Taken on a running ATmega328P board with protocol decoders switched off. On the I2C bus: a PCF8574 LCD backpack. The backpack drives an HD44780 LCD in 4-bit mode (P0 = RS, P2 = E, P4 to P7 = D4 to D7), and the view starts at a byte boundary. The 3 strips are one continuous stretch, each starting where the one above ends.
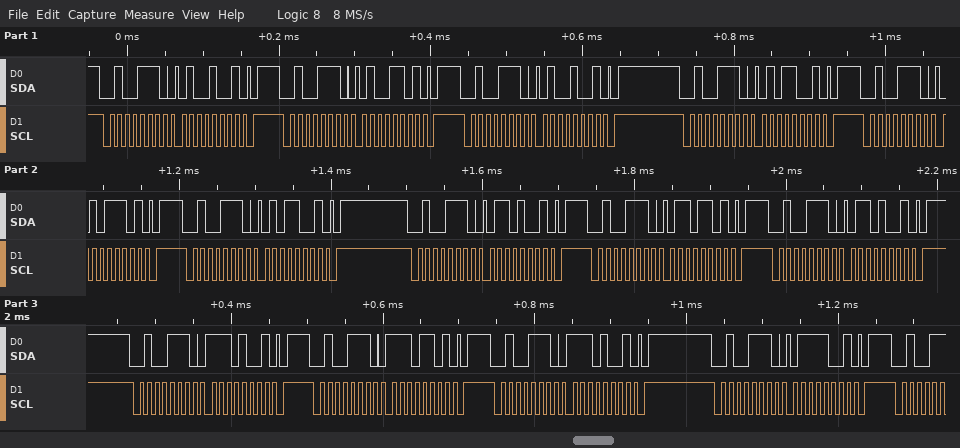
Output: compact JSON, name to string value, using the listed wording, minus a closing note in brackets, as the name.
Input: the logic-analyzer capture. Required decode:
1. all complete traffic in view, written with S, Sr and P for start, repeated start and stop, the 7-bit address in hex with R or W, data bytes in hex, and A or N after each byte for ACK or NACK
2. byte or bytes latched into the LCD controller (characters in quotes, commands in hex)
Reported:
{"all complete traffic in view, written with S, Sr and P for start, repeated start and stop, the 7-bit address in hex with R or W, data bytes in hex, and A or N after each byte for ACK or NACK": "S 27W A 49 A P S 27W A 4D A P S 27W A 49 A P S 27W A 59 A P S 27W A 5D A P S 27W A 59 A P S 27W A 69 A P S 27W A 6D A P S 27W A 69 A P S 27W A E9 A P S 27W A ED A P S 27W A E9 A P S 27W A 79 A P", "byte or bytes latched into the LCD controller": "'E' 'n'"}
